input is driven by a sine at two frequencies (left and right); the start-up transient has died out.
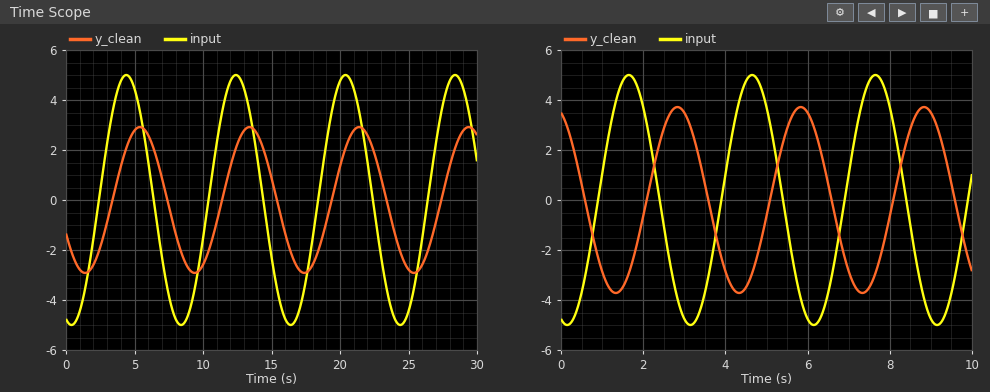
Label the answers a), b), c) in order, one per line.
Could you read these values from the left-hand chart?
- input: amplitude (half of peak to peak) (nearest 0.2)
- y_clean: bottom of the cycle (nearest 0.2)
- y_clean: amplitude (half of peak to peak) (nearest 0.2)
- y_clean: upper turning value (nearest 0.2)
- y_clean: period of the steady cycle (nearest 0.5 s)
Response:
a) 5.0
b) -3.0
c) 3.0
d) 3.0
e) 8.0 s
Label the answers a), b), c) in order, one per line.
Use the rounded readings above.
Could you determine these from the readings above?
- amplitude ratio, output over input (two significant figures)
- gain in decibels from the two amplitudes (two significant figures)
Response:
a) 0.60
b) -4.4 dB
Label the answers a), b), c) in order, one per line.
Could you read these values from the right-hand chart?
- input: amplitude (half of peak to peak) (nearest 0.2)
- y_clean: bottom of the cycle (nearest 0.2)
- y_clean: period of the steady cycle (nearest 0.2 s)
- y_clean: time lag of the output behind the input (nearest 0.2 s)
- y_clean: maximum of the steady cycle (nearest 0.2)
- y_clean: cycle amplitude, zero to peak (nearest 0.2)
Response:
a) 5.0
b) -3.8
c) 3.0 s
d) 1.2 s
e) 3.8
f) 3.8
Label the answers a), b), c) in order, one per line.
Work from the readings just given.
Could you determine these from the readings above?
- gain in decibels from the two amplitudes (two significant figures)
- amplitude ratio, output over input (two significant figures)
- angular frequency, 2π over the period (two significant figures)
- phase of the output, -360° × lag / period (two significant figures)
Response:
a) -2.4 dB
b) 0.76
c) 2.1 rad/s
d) -140°
